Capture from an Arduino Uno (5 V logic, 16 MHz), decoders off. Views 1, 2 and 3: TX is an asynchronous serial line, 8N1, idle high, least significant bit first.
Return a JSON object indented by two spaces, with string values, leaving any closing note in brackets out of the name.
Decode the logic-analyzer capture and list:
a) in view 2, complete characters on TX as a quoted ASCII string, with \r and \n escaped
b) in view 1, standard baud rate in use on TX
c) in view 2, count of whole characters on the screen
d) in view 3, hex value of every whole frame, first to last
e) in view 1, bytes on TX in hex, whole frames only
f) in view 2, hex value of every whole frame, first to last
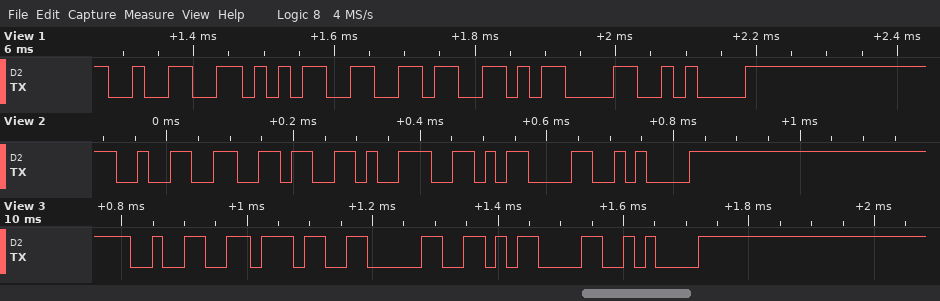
{
  "in view 2, complete characters on TX as a quoted ASCII string, with \\r and \\n escaped": "\"269\\r\\n\"",
  "in view 1, standard baud rate in use on TX": "57600 baud",
  "in view 2, count of whole characters on the screen": "5",
  "in view 3, hex value of every whole frame, first to last": "32 37 30 0D 0A",
  "in view 1, bytes on TX in hex, whole frames only": "0x32 0x35 0x36 0x0D 0x0A",
  "in view 2, hex value of every whole frame, first to last": "0x32 0x36 0x39 0x0D 0x0A"
}
